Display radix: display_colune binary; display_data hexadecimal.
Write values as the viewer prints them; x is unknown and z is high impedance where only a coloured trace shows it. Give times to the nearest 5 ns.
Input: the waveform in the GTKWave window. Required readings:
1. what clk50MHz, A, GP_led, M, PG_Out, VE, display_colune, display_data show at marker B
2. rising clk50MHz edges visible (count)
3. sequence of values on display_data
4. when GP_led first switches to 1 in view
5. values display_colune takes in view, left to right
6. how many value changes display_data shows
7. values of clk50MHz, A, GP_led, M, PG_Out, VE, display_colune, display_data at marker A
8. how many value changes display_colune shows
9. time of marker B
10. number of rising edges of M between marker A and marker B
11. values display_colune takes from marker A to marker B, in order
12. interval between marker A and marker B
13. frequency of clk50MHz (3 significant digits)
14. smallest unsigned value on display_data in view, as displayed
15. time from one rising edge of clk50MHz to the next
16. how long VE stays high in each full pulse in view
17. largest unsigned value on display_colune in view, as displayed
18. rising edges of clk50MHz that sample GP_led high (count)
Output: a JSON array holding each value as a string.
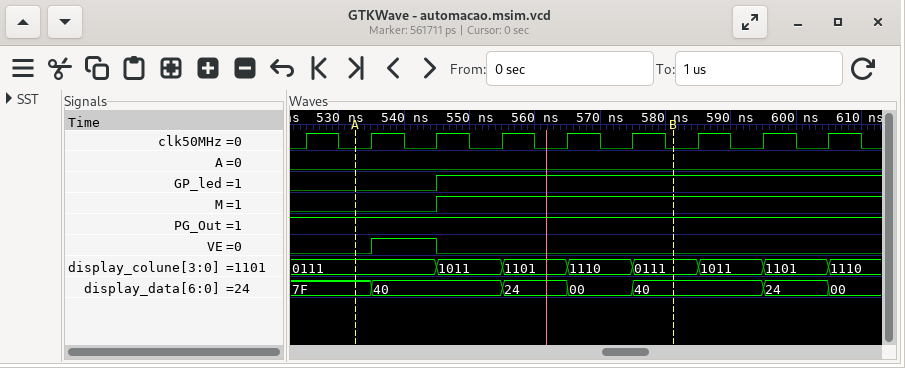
["clk50MHz=0, A=0, GP_led=1, M=1, PG_Out=1, VE=0, display_colune=0111, display_data=40", "9", "7F, 40, 24, 00, 40, 24, 00", "545 ns", "0111, 1011, 1101, 1110, 0111, 1011, 1101, 1110", "6", "clk50MHz=0, A=0, GP_led=0, M=0, PG_Out=1, VE=0, display_colune=0111, display_data=7F", "7", "580 ns", "1", "0111, 1011, 1101, 1110, 0111", "50 ns", "100 MHz", "00", "10 ns", "10 ns", "1110", "6"]
